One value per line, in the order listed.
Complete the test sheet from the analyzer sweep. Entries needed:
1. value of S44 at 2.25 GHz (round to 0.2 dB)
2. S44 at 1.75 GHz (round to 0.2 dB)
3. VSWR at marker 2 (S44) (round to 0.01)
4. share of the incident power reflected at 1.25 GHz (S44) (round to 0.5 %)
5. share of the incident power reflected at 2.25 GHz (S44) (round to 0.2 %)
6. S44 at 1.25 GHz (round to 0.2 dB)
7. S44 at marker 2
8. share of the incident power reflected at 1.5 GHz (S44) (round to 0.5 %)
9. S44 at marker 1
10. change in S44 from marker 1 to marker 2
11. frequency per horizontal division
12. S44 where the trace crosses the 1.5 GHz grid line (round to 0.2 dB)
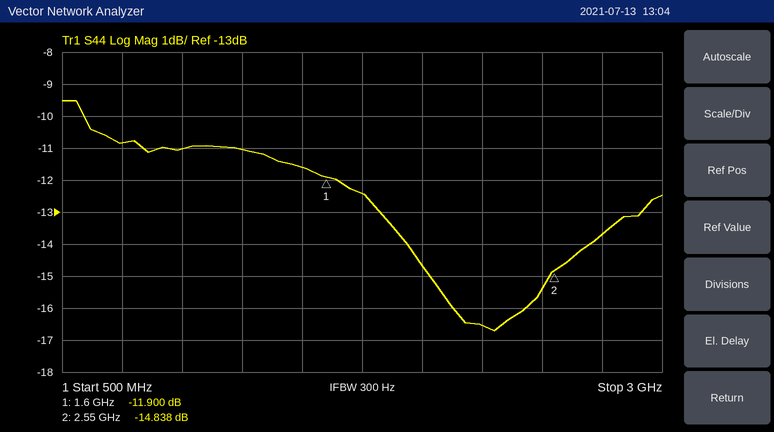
-16.6 dB
-12.4 dB
1.44
8.0 %
2.2 %
-11.0 dB
-14.838 dB
7.0 %
-11.900 dB
-2.938 dB
250 MHz
-11.6 dB
